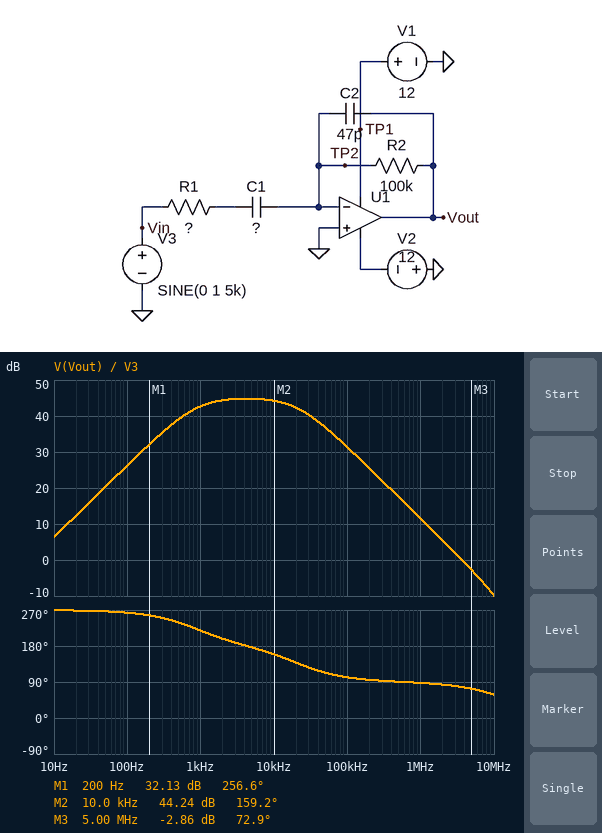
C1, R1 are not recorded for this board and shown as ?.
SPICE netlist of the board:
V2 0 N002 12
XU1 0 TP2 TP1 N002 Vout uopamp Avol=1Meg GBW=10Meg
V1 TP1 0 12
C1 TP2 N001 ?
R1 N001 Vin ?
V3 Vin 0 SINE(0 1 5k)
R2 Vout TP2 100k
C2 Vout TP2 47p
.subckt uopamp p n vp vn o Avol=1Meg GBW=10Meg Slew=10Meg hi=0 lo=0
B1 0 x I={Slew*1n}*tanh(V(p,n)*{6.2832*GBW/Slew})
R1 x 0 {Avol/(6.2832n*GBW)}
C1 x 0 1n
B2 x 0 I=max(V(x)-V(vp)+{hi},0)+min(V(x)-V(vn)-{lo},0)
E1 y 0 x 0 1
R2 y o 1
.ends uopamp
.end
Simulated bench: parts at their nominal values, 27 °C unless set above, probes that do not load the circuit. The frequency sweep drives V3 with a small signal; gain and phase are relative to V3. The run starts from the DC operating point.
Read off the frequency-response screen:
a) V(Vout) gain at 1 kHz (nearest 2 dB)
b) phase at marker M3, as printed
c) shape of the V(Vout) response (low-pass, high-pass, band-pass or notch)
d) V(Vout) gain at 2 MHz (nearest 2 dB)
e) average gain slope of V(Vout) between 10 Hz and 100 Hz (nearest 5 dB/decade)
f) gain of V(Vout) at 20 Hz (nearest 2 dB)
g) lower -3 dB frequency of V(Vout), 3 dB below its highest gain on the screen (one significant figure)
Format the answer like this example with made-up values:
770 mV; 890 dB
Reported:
42 dB; 72.9 deg; band-pass; 6 dB; 20 dB/decade; 12 dB; 800 Hz
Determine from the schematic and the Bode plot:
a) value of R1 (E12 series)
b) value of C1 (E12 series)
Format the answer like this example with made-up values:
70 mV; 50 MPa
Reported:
560 Ω; 330 nF
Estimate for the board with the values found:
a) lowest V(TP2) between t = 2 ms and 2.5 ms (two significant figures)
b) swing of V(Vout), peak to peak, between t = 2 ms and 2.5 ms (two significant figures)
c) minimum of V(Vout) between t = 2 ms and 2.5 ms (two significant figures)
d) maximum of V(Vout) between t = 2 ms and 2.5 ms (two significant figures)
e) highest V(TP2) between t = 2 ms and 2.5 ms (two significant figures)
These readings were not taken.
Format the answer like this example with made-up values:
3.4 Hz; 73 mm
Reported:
-940 mV; 24 V; -12 V; 12 V; 920 mV
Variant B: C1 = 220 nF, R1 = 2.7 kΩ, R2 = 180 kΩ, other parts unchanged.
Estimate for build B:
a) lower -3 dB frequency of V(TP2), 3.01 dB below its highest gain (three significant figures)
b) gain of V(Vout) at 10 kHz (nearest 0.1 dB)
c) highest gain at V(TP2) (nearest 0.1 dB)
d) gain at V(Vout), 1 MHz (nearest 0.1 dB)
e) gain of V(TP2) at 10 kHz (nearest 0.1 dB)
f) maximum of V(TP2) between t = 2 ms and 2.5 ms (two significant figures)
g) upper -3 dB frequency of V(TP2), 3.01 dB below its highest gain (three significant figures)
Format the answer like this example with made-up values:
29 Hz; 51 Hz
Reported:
16.6 kHz; 35.2 dB; -19.1 dB; 0.9 dB; -24.8 dB; 800 mV; 11.3 MHz
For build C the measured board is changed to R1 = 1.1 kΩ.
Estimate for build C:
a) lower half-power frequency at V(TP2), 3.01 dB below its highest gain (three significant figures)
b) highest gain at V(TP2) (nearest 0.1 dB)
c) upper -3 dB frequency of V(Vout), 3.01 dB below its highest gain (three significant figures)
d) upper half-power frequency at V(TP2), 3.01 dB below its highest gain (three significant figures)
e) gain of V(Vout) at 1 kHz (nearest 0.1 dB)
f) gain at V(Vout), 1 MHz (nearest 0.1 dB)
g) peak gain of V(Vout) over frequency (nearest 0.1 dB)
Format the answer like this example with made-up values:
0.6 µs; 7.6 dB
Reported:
25.7 kHz; -12.6 dB; 26.6 kHz; 13.1 MHz; 38.4 dB; 7.4 dB; 39.1 dB
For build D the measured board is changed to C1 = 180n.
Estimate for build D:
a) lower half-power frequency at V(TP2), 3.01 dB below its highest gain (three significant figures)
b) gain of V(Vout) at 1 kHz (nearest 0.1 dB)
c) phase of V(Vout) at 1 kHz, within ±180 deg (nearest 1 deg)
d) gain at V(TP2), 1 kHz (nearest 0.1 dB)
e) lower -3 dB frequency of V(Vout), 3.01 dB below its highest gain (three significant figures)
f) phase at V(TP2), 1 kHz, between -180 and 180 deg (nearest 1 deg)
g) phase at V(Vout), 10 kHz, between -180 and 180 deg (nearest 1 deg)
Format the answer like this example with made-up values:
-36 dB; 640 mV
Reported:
20.5 kHz; 39.7 dB; -124 deg; -40.3 dB; 1.42 kHz; 145 deg; 163 deg
